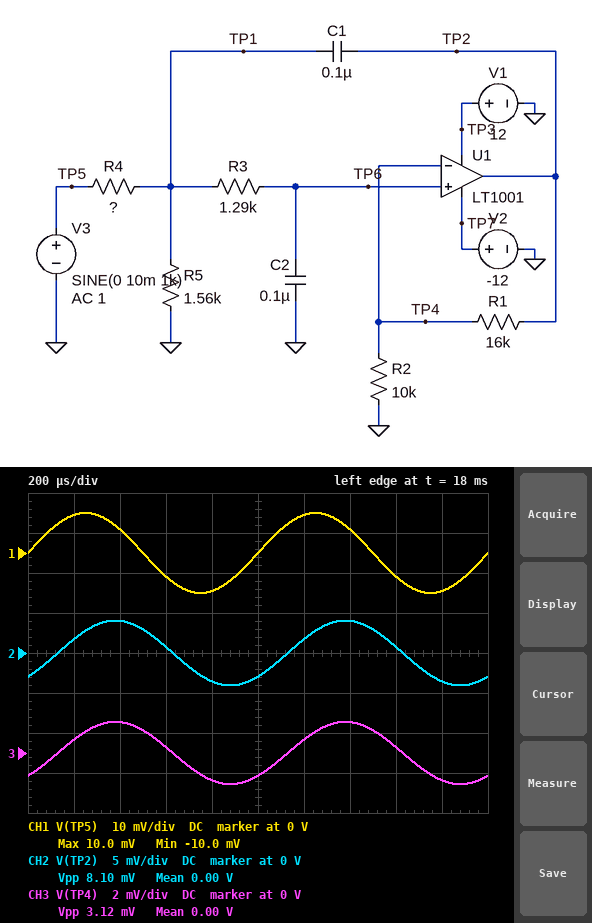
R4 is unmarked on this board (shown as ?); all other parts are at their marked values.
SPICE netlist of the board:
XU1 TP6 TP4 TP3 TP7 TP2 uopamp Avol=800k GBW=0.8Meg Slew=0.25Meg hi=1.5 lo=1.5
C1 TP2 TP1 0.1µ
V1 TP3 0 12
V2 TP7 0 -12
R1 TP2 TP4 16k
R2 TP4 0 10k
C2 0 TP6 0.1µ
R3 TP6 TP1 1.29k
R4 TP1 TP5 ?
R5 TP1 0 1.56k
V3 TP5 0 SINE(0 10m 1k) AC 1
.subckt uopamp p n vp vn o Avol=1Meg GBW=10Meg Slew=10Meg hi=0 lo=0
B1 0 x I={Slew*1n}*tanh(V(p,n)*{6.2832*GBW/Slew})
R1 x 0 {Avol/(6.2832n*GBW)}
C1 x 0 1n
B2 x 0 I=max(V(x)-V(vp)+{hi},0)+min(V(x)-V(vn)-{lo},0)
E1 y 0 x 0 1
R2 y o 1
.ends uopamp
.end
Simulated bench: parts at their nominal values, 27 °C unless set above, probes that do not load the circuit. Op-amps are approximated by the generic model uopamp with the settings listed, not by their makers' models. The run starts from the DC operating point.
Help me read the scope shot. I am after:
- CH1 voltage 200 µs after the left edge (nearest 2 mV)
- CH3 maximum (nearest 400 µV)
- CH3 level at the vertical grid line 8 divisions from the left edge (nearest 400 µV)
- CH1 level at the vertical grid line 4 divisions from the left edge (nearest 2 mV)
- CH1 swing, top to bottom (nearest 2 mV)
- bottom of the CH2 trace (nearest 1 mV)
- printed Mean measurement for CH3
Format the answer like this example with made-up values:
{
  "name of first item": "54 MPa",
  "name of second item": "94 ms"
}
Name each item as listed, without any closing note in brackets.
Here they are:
{
  "CH1 voltage 200 µs after the left edge": "10 mV",
  "CH3 maximum": "1.6 mV",
  "CH3 level at the vertical grid line 8 divisions from the left edge": "400 µV",
  "CH1 level at the vertical grid line 4 divisions from the left edge": "-10 mV",
  "CH1 swing, top to bottom": "20 mV",
  "bottom of the CH2 trace": "-4 mV",
  "printed Mean measurement for CH3": "0.00 V"
}
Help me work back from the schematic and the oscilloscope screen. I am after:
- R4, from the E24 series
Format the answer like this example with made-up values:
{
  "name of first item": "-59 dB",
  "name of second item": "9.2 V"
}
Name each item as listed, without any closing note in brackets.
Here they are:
{
  "R4, from the E24 series": "27 kΩ"
}
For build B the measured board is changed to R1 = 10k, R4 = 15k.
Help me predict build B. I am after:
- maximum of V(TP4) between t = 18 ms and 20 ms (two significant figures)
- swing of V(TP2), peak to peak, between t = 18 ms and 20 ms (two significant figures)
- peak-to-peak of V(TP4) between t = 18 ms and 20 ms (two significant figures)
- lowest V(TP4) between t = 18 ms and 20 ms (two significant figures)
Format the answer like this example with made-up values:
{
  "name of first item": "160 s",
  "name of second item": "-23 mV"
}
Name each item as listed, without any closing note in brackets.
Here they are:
{
  "maximum of V(TP4) between t = 18 ms and 20 ms": "1.1 mV",
  "swing of V(TP2), peak to peak, between t = 18 ms and 20 ms": "4.4 mV",
  "peak-to-peak of V(TP4) between t = 18 ms and 20 ms": "2.2 mV",
  "lowest V(TP4) between t = 18 ms and 20 ms": "-1.1 mV"
}
